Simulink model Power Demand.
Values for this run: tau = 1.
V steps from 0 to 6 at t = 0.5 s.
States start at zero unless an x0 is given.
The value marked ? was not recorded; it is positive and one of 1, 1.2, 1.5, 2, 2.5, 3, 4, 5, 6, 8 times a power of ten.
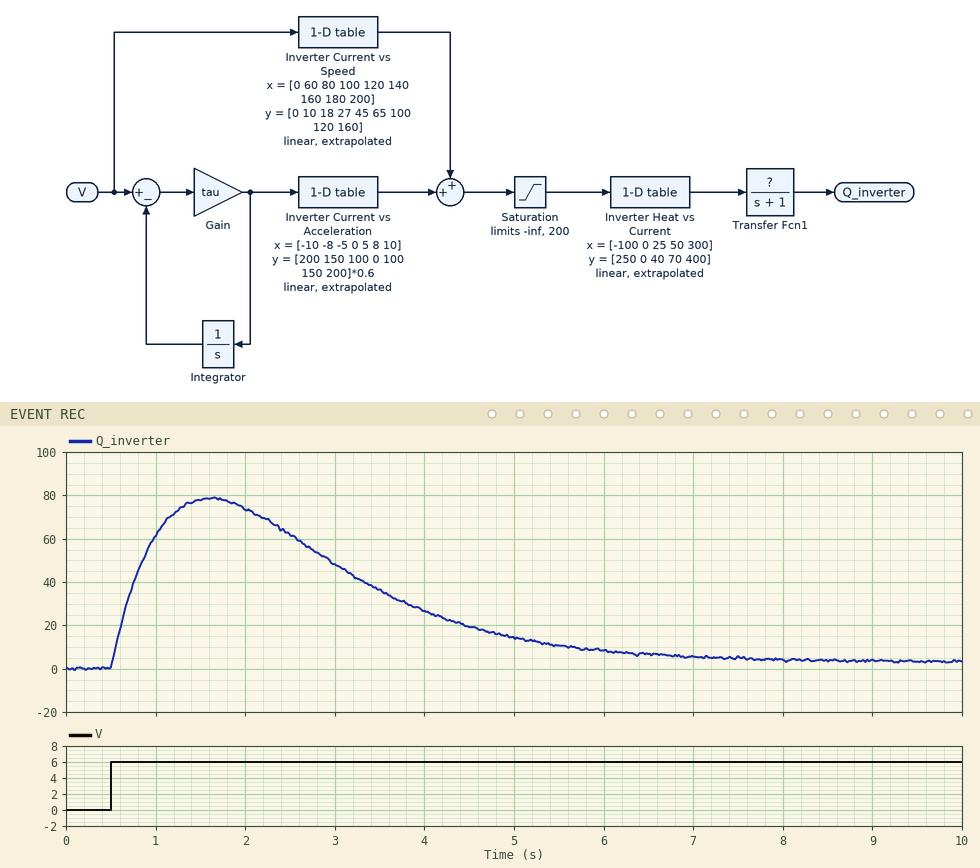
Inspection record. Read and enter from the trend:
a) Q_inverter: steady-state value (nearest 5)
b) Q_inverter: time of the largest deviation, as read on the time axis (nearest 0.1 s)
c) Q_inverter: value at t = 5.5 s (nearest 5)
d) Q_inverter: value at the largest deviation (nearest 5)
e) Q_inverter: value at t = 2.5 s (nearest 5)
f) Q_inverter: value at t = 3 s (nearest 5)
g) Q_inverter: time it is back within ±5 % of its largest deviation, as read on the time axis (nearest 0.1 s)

5
1.6 s
10
80
60
50
6.3 s
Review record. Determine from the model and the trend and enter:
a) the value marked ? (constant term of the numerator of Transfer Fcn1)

2
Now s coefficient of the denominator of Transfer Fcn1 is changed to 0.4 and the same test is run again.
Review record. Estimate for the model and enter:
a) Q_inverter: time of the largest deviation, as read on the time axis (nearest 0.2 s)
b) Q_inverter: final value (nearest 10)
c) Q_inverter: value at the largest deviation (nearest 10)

1.2 s
0
110
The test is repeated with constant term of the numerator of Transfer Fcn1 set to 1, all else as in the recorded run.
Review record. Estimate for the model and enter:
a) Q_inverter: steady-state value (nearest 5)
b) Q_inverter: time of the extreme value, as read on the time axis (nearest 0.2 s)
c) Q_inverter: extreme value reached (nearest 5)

0
1.6 s
40
